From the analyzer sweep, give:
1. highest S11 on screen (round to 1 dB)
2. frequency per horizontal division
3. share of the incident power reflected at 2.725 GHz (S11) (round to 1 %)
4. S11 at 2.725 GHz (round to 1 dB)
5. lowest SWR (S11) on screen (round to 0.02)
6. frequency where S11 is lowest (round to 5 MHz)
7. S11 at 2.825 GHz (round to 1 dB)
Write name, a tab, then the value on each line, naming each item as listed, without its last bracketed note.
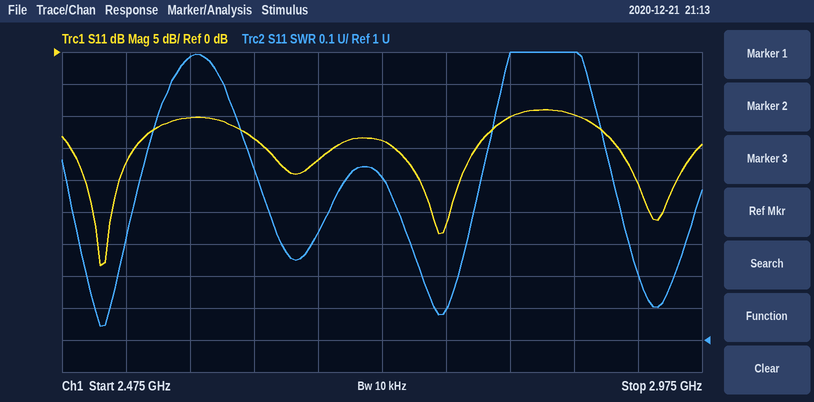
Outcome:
highest S11 on screen	-9 dB
frequency per horizontal division	50 MHz
share of the incident power reflected at 2.725 GHz (S11)	4 %
S11 at 2.725 GHz	-14 dB
lowest SWR (S11) on screen	1.04
frequency where S11 is lowest	2.505 GHz
S11 at 2.825 GHz	-10 dB
